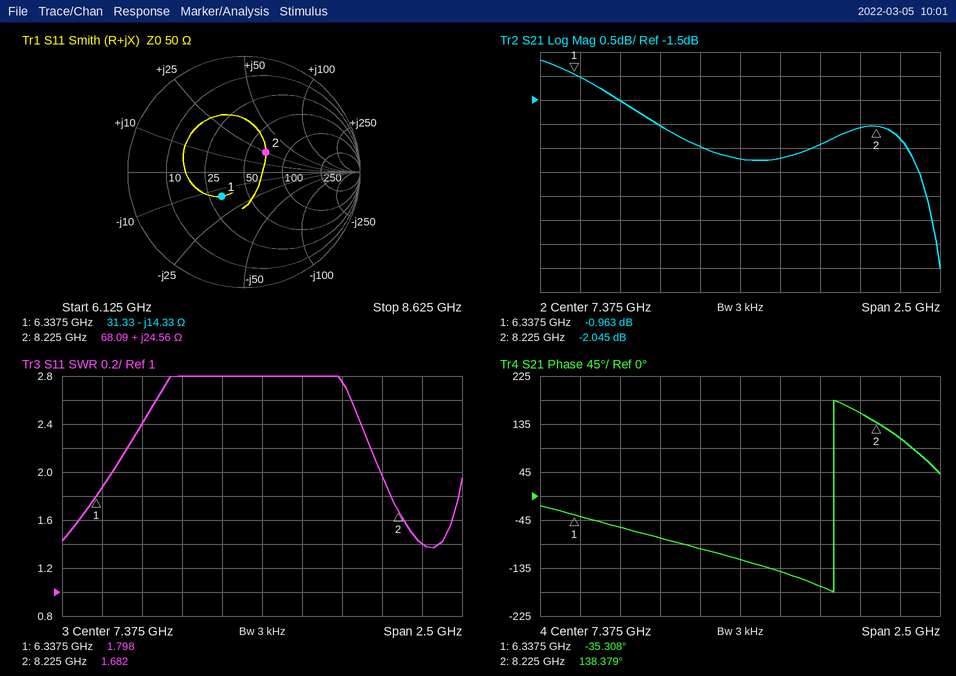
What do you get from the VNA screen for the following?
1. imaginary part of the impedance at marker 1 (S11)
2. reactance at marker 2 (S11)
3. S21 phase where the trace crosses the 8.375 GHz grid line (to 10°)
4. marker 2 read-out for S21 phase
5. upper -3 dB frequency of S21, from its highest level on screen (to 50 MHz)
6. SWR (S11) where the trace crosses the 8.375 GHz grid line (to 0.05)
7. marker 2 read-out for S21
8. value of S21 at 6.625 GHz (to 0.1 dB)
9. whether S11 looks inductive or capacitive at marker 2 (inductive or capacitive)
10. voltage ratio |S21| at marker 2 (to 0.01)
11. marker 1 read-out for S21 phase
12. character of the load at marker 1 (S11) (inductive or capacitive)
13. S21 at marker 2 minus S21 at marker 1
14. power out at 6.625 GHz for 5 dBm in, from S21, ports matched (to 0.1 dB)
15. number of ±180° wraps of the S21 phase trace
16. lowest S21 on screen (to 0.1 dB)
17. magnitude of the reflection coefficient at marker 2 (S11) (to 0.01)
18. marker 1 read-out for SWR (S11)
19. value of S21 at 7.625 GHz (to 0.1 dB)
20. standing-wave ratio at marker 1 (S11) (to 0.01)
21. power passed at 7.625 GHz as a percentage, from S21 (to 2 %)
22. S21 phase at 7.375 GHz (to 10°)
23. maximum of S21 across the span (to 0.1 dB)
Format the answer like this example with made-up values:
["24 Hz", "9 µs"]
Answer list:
["-14.33 Ω", "+24.56 Ω", "110°", "138.379°", "8.55 GHz", "1.40", "-2.045 dB", "-1.5 dB", "inductive", "0.79", "-35.308°", "capacitive", "-1.082 dB", "3.5 dBm", "1", "-5.0 dB", "0.25", "1.798", "-2.7 dB", "1.80", "54 %", "-120°", "-0.7 dB"]
